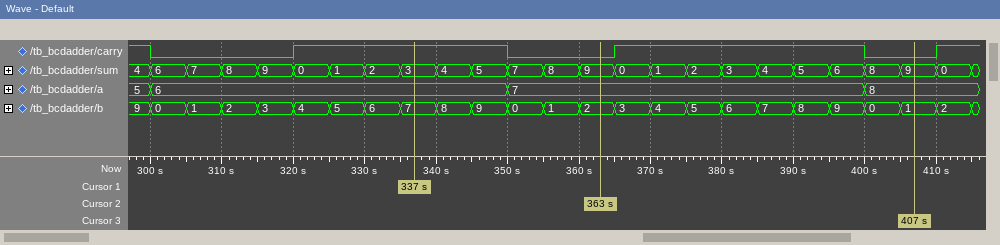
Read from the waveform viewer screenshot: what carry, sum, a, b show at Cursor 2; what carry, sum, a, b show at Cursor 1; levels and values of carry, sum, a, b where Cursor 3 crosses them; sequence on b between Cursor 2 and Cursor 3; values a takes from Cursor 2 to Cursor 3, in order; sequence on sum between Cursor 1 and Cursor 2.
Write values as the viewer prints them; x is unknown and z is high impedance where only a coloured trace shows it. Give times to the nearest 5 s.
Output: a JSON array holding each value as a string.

["carry=0, sum=9, a=7, b=2", "carry=1, sum=3, a=6, b=7", "carry=0, sum=9, a=8, b=1", "2, 3, 4, 5, 6, 7, 8, 9, 0, 1", "7, 8", "3, 4, 5, 7, 8, 9"]
